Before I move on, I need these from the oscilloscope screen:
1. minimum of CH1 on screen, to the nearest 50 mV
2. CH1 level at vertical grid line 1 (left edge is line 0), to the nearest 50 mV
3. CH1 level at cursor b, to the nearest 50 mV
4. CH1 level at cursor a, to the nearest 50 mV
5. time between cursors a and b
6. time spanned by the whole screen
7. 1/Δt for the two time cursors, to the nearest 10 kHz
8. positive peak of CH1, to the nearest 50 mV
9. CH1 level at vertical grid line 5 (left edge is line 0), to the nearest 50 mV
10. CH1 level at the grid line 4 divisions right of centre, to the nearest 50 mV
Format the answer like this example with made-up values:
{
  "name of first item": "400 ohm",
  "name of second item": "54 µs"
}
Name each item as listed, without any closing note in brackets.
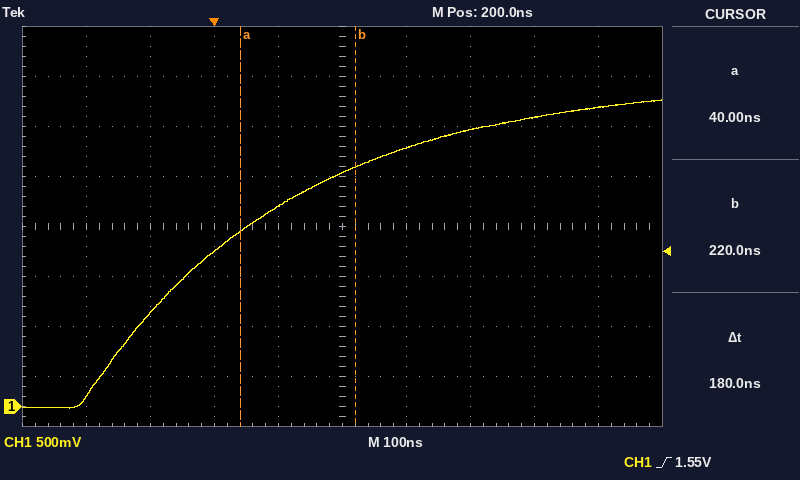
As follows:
{
  "minimum of CH1 on screen, to the nearest 50 mV": "0 mV",
  "CH1 level at vertical grid line 1 (left edge is line 0), to the nearest 50 mV": "100 mV",
  "CH1 level at cursor b, to the nearest 50 mV": "2.40 V",
  "CH1 level at cursor a, to the nearest 50 mV": "1.75 V",
  "time between cursors a and b": "180 ns",
  "time spanned by the whole screen": "1 µs",
  "1/Δt for the two time cursors, to the nearest 10 kHz": "5.56 MHz",
  "positive peak of CH1, to the nearest 50 mV": "3.05 V",
  "CH1 level at vertical grid line 5 (left edge is line 0), to the nearest 50 mV": "2.35 V",
  "CH1 level at the grid line 4 divisions right of centre, to the nearest 50 mV": "3.00 V"
}
